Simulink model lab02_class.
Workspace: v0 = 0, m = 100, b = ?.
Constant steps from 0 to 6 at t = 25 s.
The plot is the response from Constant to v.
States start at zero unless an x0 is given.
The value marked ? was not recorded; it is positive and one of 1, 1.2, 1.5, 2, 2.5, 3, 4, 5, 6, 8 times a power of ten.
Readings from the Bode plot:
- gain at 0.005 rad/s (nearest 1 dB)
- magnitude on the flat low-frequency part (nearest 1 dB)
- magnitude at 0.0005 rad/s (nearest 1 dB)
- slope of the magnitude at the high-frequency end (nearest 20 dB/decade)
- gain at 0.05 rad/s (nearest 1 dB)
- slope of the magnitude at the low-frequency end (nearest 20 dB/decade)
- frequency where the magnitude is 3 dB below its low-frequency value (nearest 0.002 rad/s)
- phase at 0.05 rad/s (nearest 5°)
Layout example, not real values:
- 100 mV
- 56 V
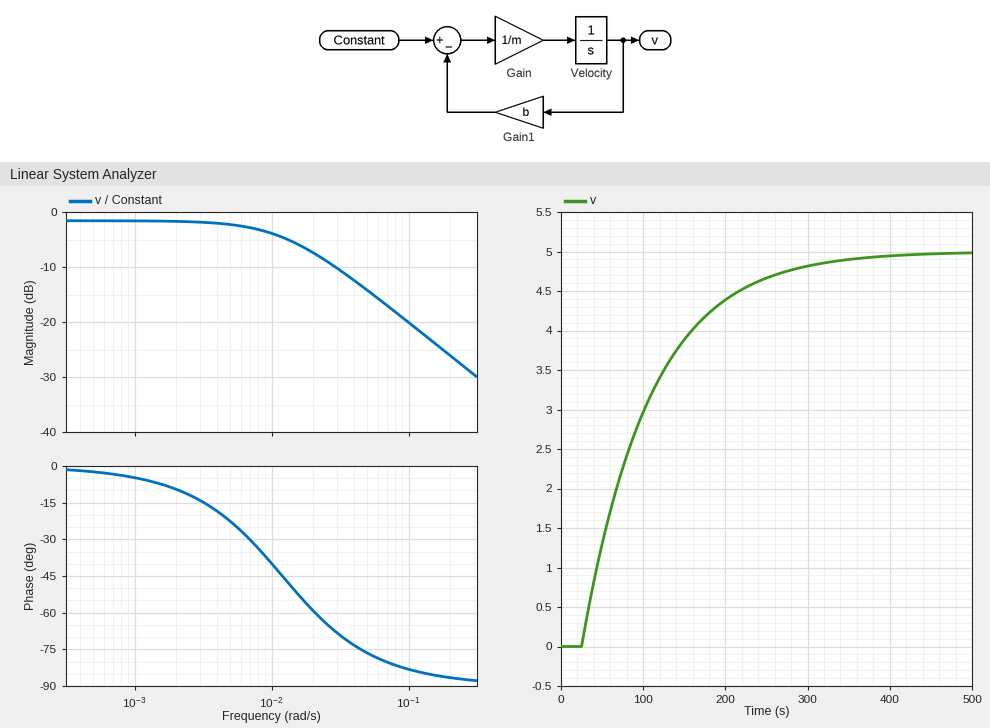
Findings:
- -2 dB
- -2 dB
- -2 dB
- -20 dB/decade
- -14 dB
- 0 dB/decade
- 0.012 rad/s
- -75°
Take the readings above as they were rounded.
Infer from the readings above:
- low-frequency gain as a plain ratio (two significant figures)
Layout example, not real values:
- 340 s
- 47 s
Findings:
- 0.79
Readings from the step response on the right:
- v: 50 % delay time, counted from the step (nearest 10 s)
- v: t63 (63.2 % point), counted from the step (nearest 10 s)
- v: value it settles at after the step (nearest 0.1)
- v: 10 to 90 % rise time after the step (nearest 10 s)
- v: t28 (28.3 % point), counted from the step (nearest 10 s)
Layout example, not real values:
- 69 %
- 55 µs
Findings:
- 60 s
- 80 s
- 5.0
- 180 s
- 30 s
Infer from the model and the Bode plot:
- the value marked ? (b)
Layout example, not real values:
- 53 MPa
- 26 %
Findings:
- 1.2
